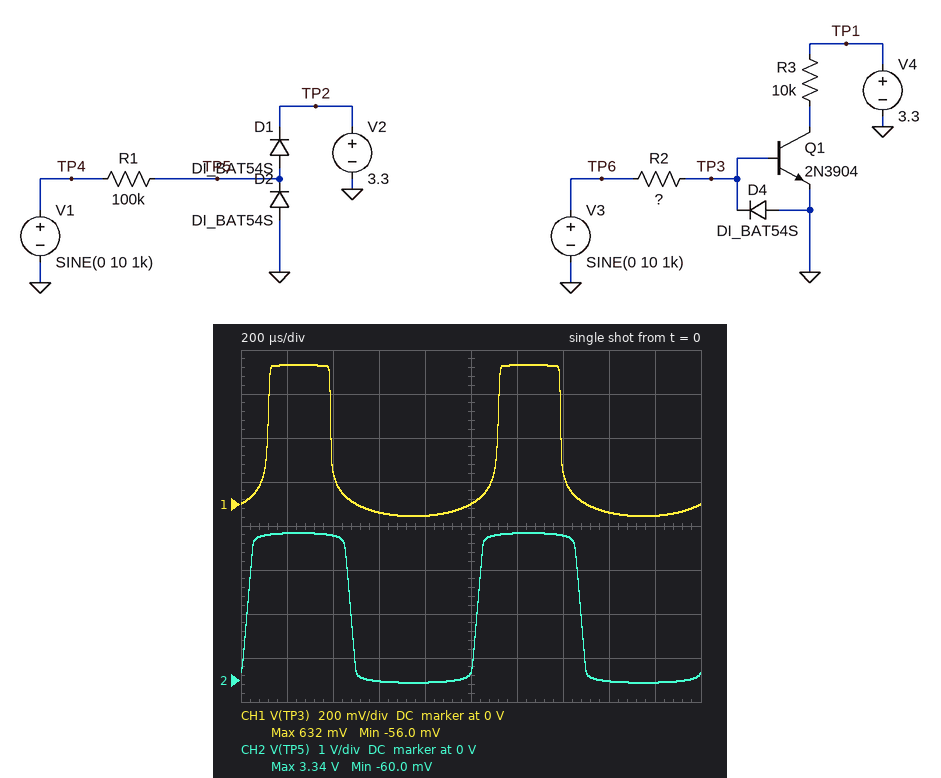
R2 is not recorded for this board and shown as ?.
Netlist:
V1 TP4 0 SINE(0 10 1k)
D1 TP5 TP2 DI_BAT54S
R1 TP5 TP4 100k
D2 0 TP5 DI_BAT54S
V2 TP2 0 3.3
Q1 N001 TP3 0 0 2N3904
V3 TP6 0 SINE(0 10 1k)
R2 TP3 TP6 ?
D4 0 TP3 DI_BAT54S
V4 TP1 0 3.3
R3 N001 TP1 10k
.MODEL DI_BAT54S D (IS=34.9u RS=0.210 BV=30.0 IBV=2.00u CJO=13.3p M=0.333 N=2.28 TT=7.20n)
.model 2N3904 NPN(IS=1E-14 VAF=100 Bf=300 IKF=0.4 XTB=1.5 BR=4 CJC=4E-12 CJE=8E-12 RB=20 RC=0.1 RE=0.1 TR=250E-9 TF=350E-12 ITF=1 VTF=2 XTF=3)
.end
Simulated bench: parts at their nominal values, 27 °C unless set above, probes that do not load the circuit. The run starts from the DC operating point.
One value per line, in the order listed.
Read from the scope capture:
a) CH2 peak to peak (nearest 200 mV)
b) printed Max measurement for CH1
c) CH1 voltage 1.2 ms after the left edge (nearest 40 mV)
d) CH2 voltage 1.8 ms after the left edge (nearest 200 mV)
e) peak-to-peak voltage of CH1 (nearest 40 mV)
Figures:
3.4 V
632 mV
640 mV
0 V
680 mV
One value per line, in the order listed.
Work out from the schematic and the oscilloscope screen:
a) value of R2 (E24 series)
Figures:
180 kΩ
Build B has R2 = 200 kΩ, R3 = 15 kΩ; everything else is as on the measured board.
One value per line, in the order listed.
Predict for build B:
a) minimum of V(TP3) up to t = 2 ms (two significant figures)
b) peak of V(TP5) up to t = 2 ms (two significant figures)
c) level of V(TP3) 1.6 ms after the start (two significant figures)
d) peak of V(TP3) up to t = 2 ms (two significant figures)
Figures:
-52 mV
3.3 V
-36 mV
620 mV
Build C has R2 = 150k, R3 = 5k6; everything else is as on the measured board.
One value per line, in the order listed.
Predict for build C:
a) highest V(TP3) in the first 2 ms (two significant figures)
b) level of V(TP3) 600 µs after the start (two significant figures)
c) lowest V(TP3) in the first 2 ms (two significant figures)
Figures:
650 mV
-44 mV
-63 mV
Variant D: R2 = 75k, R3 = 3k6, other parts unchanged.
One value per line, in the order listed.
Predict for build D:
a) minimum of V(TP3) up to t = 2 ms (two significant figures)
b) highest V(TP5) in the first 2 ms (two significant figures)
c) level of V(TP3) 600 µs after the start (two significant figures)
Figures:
-92 mV
3.3 V
-69 mV
